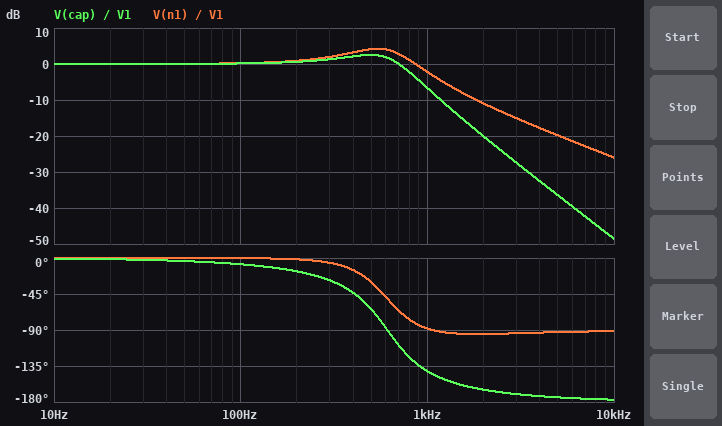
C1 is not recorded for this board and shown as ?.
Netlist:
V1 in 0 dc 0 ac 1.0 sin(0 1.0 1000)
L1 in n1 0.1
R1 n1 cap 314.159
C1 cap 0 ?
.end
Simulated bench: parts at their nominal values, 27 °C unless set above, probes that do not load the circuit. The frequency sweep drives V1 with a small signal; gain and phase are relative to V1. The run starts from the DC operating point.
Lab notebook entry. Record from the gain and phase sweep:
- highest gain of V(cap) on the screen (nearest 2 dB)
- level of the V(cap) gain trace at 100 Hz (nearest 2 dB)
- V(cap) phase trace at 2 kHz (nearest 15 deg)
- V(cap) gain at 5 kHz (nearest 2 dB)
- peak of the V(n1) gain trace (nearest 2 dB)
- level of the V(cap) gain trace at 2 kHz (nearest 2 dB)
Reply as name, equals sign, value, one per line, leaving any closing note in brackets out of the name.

highest gain of V(cap) on the screen = 2 dB
level of the V(cap) gain trace at 100 Hz = 0 dB
V(cap) phase trace at 2 kHz = -165 deg
V(cap) gain at 5 kHz = -36 dB
peak of the V(n1) gain trace = 4 dB
level of the V(cap) gain trace at 2 kHz = -20 dB
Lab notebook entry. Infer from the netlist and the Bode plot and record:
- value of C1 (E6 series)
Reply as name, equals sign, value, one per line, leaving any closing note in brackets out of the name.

value of C1 = 680 nF
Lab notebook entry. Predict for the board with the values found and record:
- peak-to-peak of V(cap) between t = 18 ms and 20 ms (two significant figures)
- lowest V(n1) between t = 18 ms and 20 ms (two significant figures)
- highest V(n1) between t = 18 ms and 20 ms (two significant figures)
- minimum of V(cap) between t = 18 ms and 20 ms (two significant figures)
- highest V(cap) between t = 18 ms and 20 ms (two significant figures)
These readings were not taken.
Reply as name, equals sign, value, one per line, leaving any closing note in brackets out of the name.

peak-to-peak of V(cap) between t = 18 ms and 20 ms = 930 mV
lowest V(n1) between t = 18 ms and 20 ms = -780 mV
highest V(n1) between t = 18 ms and 20 ms = 780 mV
minimum of V(cap) between t = 18 ms and 20 ms = -460 mV
highest V(cap) between t = 18 ms and 20 ms = 460 mV
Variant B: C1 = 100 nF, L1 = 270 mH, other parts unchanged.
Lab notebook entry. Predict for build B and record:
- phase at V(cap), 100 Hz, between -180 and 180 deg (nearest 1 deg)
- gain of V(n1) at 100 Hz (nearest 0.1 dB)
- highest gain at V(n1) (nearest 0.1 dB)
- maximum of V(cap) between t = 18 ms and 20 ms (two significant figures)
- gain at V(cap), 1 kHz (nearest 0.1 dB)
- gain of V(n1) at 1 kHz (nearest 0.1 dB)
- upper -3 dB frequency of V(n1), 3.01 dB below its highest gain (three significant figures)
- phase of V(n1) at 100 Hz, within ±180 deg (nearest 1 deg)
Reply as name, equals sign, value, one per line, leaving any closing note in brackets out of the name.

phase at V(cap), 100 Hz, between -180 and 180 deg = -1 deg
gain of V(n1) at 100 Hz = 0.1 dB
highest gain at V(n1) = 14.6 dB
maximum of V(cap) between t = 18 ms and 20 ms = 4.8 V
gain at V(cap), 1 kHz = 13.6 dB
gain of V(n1) at 1 kHz = 13.8 dB
upper -3 dB frequency of V(n1), 3.01 dB below its highest gain = 1.05 kHz
phase of V(n1) at 100 Hz, within ±180 deg = 0 deg
